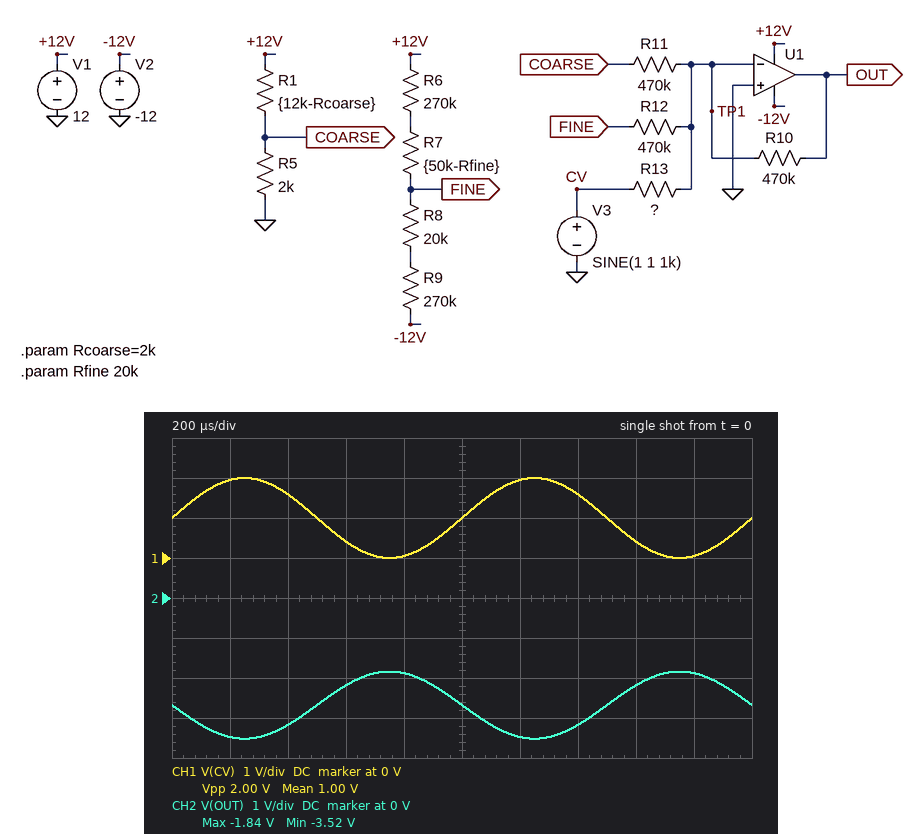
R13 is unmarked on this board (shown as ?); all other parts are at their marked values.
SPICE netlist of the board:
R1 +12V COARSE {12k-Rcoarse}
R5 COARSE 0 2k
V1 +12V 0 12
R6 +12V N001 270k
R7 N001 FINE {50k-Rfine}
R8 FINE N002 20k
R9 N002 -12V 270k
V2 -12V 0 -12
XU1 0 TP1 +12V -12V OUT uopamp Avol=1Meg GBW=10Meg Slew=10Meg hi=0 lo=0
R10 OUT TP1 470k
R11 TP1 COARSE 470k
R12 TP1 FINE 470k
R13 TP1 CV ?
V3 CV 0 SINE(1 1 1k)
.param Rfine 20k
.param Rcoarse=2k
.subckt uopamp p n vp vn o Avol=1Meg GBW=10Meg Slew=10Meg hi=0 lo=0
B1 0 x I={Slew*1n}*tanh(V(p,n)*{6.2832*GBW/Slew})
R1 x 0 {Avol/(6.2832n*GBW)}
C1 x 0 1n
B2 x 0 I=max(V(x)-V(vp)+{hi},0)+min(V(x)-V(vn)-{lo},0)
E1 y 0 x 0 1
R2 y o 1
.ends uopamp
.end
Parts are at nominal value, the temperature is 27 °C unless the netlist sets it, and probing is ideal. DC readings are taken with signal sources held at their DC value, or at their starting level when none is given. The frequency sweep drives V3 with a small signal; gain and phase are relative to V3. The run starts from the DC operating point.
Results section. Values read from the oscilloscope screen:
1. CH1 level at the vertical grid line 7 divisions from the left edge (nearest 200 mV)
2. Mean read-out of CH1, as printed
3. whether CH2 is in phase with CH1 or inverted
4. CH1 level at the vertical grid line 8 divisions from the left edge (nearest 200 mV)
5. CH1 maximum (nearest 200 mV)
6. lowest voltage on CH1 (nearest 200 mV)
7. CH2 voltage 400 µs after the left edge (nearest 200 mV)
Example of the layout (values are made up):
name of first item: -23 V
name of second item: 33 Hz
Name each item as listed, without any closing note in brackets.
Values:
CH1 level at the vertical grid line 7 divisions from the left edge: 1.6 V
Mean read-out of CH1, as printed: 1.00 V
whether CH2 is in phase with CH1 or inverted: inverted
CH1 level at the vertical grid line 8 divisions from the left edge: 400 mV
CH1 maximum: 2.0 V
lowest voltage on CH1: 0 V
CH2 voltage 400 µs after the left edge: -3.2 V
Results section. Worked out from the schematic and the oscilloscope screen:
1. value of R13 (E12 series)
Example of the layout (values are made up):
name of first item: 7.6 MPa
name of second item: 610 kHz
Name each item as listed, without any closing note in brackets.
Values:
value of R13: 560 kΩ
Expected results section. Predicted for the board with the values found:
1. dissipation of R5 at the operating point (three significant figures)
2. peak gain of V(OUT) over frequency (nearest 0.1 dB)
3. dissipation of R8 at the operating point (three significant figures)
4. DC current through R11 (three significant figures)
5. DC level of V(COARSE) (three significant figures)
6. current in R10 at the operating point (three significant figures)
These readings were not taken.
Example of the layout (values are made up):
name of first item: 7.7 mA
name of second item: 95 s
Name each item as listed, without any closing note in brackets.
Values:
dissipation of R5 at the operating point: 1.99 mW
peak gain of V(OUT) over frequency: -1.5 dB
dissipation of R8 at the operating point: 33.4 µW
DC current through R11: 4.24 µA
DC level of V(COARSE): 1.99 V
current in R10 at the operating point: 5.70 µA
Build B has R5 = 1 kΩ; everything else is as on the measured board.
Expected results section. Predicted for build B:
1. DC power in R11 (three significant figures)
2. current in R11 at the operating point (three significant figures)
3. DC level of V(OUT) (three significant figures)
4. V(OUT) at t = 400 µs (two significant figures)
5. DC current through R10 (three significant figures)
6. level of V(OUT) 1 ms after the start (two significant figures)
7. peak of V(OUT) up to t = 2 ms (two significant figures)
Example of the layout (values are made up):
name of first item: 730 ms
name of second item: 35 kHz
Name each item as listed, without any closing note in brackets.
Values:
DC power in R11: 2.52 µW
current in R11 at the operating point: 2.32 µA
DC level of V(OUT): -1.77 V
V(OUT) at t = 400 µs: -2.3 V
DC current through R10: 3.77 µA
level of V(OUT) 1 ms after the start: -1.8 V
peak of V(OUT) up to t = 2 ms: -930 mV
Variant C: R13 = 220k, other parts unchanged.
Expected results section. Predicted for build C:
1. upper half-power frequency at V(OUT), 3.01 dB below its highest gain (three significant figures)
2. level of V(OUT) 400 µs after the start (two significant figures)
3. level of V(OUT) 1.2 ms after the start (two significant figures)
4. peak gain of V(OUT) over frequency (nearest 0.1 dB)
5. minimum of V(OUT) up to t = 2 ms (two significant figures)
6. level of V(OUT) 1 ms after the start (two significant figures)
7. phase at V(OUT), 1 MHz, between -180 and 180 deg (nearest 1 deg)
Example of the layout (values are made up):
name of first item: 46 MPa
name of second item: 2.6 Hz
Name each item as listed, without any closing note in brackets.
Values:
upper half-power frequency at V(OUT), 3.01 dB below its highest gain: 2.04 MHz
level of V(OUT) 400 µs after the start: -5.2 V
level of V(OUT) 1.2 ms after the start: -6.0 V
peak gain of V(OUT) over frequency: 6.6 dB
minimum of V(OUT) up to t = 2 ms: -6.1 V
level of V(OUT) 1 ms after the start: -4.0 V
phase at V(OUT), 1 MHz, between -180 and 180 deg: 154 deg
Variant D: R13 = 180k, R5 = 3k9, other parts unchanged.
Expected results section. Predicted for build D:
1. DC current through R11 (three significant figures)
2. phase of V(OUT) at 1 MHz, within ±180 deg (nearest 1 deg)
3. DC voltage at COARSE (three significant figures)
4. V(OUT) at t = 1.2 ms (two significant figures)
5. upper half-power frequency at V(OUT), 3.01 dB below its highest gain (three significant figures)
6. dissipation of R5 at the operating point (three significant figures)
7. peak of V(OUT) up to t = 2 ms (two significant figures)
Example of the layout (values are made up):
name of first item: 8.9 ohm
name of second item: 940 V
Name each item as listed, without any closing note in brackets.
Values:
DC current through R11: 7.12 µA
phase of V(OUT) at 1 MHz, within ±180 deg: 152 deg
DC voltage at COARSE: 3.35 V
V(OUT) at t = 1.2 ms: -8.3 V
upper half-power frequency at V(OUT), 3.01 dB below its highest gain: 1.86 MHz
dissipation of R5 at the operating point: 2.87 mW
peak of V(OUT) up to t = 2 ms: -3.2 V
